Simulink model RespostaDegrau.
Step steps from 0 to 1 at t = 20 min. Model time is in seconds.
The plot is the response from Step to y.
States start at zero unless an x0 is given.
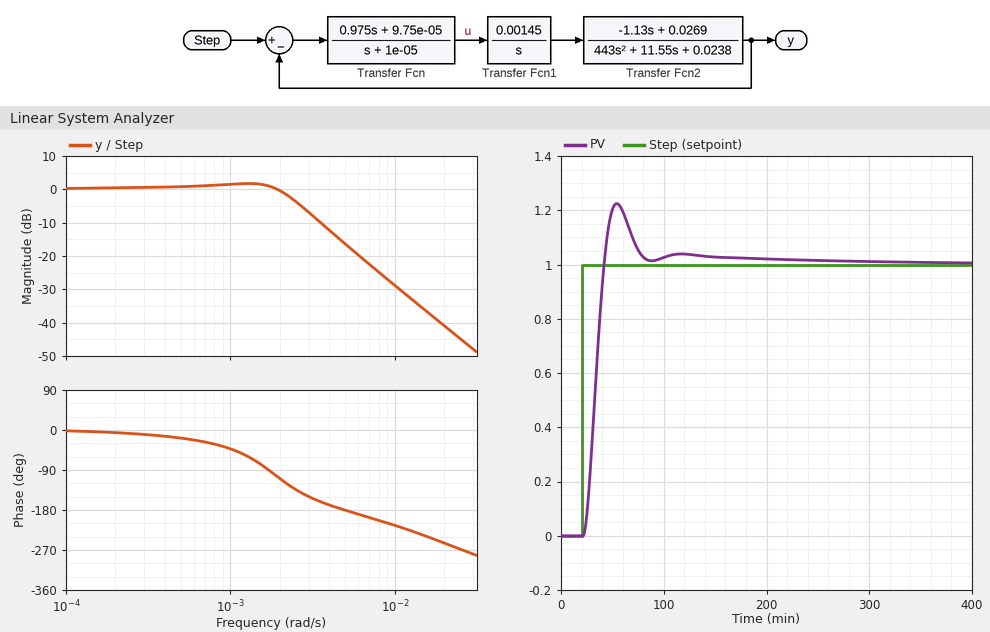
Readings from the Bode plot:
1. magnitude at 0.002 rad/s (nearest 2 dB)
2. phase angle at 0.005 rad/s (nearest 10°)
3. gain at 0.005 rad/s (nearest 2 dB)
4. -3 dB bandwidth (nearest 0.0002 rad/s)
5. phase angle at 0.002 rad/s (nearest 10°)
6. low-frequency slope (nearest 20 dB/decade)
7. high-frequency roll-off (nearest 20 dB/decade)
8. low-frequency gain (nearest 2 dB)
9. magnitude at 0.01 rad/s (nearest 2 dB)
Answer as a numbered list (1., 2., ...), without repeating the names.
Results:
1. 0 dB
2. -180°
3. -16 dB
4. 0.0024 rad/s
5. -110°
6. 0 dB/decade
7. -40 dB/decade
8. 0 dB
9. -28 dB
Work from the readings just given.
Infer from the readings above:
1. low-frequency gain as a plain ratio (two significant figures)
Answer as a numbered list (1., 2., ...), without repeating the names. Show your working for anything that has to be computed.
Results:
1. 10^(0 / 20) = 1.0
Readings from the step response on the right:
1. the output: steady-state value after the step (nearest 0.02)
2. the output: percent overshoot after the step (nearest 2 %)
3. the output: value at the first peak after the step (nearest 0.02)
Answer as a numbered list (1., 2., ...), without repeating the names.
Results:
1. 1.00
2. 22 %
3. 1.22
